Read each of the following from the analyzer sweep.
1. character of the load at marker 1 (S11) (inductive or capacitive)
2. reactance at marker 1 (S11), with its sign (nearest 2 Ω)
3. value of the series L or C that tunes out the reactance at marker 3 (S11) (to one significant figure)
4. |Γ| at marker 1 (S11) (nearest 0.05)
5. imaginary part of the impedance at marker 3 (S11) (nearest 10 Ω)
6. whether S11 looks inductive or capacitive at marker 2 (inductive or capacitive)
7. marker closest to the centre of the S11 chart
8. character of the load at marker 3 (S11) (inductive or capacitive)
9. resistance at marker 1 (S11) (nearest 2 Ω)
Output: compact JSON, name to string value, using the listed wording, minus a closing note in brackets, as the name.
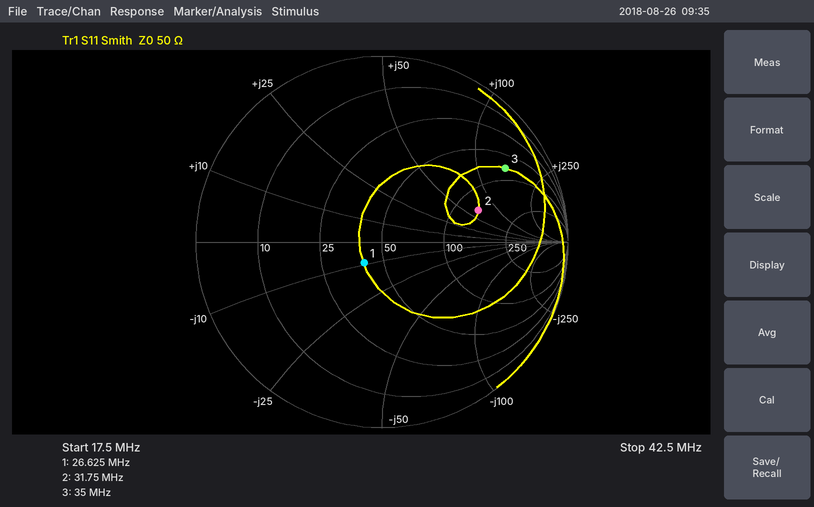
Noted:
{"character of the load at marker 1 (S11)": "capacitive", "reactance at marker 1 (S11), with its sign": "-10 Ω", "value of the series L or C that tunes out the reactance at marker 3 (S11)": "30 pF", "|Γ| at marker 1 (S11)": "0.15", "imaginary part of the impedance at marker 3 (S11)": "+150 Ω", "whether S11 looks inductive or capacitive at marker 2": "inductive", "marker closest to the centre of the S11 chart": "marker 1", "character of the load at marker 3 (S11)": "inductive", "resistance at marker 1 (S11)": "40 Ω"}
